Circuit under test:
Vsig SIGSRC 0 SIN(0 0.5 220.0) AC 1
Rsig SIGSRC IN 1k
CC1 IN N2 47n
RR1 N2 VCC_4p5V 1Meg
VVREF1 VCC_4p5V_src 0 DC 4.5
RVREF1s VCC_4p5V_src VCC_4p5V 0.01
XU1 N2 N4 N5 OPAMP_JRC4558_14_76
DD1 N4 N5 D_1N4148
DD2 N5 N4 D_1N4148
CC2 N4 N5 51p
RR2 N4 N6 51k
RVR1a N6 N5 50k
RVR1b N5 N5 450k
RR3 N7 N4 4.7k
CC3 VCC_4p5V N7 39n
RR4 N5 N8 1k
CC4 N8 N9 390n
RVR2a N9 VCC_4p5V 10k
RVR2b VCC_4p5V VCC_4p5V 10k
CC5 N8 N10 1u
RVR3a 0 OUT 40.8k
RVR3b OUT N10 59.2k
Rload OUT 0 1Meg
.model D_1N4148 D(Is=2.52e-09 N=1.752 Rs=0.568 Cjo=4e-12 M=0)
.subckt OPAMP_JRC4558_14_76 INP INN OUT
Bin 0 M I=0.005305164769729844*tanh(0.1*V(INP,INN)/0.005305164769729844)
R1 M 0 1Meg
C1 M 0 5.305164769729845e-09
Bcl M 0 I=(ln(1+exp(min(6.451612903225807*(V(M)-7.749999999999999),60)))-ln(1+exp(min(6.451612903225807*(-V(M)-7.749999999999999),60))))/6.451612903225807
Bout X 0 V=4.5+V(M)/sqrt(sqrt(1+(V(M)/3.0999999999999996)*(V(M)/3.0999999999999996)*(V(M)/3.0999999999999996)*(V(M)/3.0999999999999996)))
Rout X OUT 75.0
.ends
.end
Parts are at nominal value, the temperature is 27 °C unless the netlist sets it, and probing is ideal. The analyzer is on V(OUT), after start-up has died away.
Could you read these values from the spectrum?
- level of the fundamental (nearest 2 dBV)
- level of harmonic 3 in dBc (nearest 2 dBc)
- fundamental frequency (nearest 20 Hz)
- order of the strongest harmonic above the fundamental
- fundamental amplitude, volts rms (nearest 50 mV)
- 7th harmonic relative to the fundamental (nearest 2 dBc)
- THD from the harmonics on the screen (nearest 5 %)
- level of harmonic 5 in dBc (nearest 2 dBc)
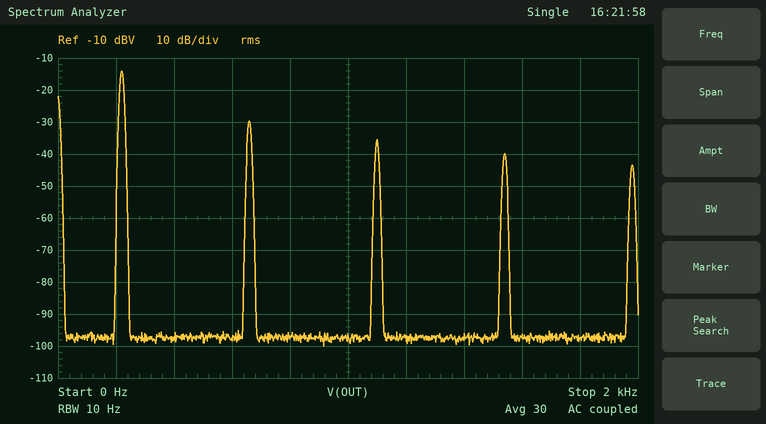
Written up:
-14 dBV
-16 dBc
220 Hz
3
200 mV
-26 dBc
20 %
-22 dBc
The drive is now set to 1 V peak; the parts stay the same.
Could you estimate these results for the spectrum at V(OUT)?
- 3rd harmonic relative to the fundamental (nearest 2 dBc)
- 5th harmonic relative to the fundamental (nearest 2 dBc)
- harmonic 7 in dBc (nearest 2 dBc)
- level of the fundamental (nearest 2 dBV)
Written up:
-18 dBc
-24 dBc
-28 dBc
-10 dBV
